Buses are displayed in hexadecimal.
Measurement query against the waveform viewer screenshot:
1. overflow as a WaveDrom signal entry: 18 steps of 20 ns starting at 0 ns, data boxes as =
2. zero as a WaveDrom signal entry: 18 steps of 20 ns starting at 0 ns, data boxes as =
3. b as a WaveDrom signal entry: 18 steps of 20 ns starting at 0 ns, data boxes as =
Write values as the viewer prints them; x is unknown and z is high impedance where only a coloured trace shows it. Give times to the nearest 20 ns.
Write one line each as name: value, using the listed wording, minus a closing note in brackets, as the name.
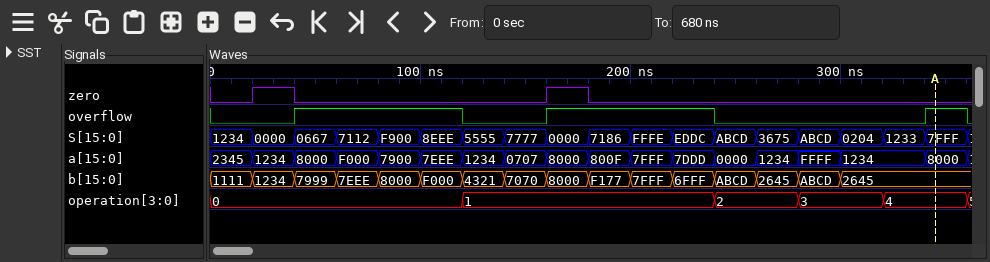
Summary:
overflow as a WaveDrom signal entry: 18 steps of 20 ns starting at 0 ns, data boxes as =: {name: 'overflow', wave: '0.1...0.1...0....1'}
zero as a WaveDrom signal entry: 18 steps of 20 ns starting at 0 ns, data boxes as =: {name: 'zero', wave: '010.....10........'}
b as a WaveDrom signal entry: 18 steps of 20 ns starting at 0 ns, data boxes as =: {name: 'b', wave: '================..', data: '1111 1234 7999 7EEE 8000 F000 4321 7070 8000 F177 7FFF 6FFF ABCD 2645 ABCD 2645'}
